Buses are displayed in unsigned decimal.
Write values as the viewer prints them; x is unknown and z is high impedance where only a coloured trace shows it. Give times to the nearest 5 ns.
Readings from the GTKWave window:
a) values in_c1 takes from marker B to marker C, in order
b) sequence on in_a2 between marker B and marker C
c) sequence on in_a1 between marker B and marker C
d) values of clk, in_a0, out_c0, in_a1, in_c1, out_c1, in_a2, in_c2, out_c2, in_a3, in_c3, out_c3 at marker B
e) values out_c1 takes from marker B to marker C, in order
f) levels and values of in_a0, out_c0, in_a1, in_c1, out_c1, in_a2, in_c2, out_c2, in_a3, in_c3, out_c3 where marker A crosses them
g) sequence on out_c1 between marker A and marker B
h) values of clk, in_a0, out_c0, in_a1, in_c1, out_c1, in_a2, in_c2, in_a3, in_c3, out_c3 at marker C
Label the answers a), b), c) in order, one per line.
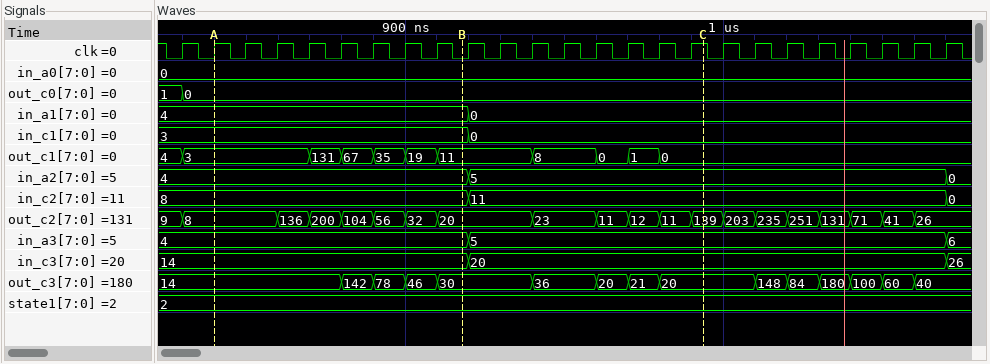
a) 3, 0
b) 4, 5
c) 4, 0
d) clk=0, in_a0=0, out_c0=0, in_a1=4, in_c1=3, out_c1=11, in_a2=4, in_c2=8, out_c2=20, in_a3=4, in_c3=14, out_c3=30
e) 11, 8, 0, 1, 0
f) in_a0=0, out_c0=0, in_a1=4, in_c1=3, out_c1=3, in_a2=4, in_c2=8, out_c2=8, in_a3=4, in_c3=14, out_c3=14
g) 3, 131, 67, 35, 19, 11
h) clk=1, in_a0=0, out_c0=0, in_a1=0, in_c1=0, out_c1=0, in_a2=5, in_c2=11, in_a3=5, in_c3=20, out_c3=20
